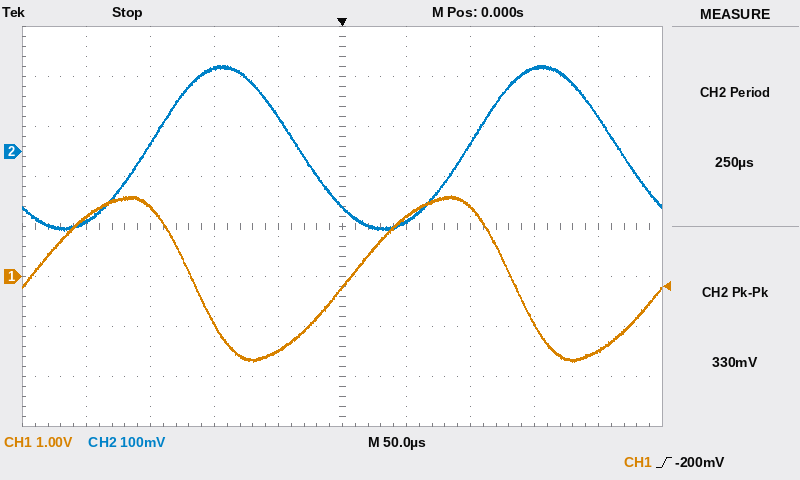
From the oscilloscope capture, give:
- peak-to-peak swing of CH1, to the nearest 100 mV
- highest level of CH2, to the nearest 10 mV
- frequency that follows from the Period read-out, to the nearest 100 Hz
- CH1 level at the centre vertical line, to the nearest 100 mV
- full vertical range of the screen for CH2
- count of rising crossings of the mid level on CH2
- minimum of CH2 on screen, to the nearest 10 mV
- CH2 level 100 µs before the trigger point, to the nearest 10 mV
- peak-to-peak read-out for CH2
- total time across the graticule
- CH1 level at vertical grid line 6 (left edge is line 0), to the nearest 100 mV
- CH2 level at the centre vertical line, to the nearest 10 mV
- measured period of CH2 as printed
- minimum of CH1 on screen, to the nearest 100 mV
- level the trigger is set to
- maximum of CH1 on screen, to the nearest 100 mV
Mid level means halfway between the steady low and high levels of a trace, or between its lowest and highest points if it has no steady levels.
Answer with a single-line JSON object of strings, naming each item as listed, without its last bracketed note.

{"peak-to-peak swing of CH1, to the nearest 100 mV": "3.3 V", "highest level of CH2, to the nearest 10 mV": "170 mV", "frequency that follows from the Period read-out, to the nearest 100 Hz": "4.0 kHz", "CH1 level at the centre vertical line, to the nearest 100 mV": "-200 mV", "full vertical range of the screen for CH2": "800 mV", "count of rising crossings of the mid level on CH2": "2", "minimum of CH2 on screen, to the nearest 10 mV": "-160 mV", "CH2 level 100 µs before the trigger point, to the nearest 10 mV": "170 mV", "peak-to-peak read-out for CH2": "330 mV", "total time across the graticule": "500 µs", "CH1 level at vertical grid line 6 (left edge is line 0), to the nearest 100 mV": "1.2 V", "CH2 level at the centre vertical line, to the nearest 10 mV": "-110 mV", "measured period of CH2 as printed": "250 µs", "minimum of CH1 on screen, to the nearest 100 mV": "-1.7 V", "level the trigger is set to": "-200 mV", "maximum of CH1 on screen, to the nearest 100 mV": "1.6 V"}
